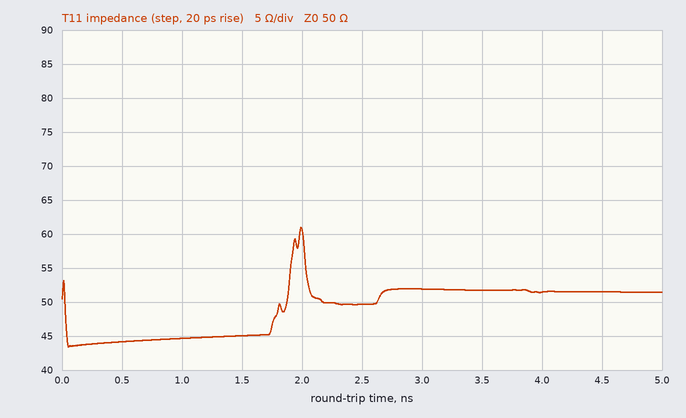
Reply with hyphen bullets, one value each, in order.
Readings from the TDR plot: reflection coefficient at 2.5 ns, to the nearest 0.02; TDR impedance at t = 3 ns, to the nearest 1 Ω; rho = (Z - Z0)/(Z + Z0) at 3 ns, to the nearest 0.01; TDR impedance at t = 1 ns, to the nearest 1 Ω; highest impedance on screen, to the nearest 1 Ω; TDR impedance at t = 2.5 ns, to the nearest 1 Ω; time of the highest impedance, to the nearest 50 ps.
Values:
- 0.00
- 52 Ω
- +0.02
- 45 Ω
- 61 Ω
- 50 Ω
- 2.00 ns
